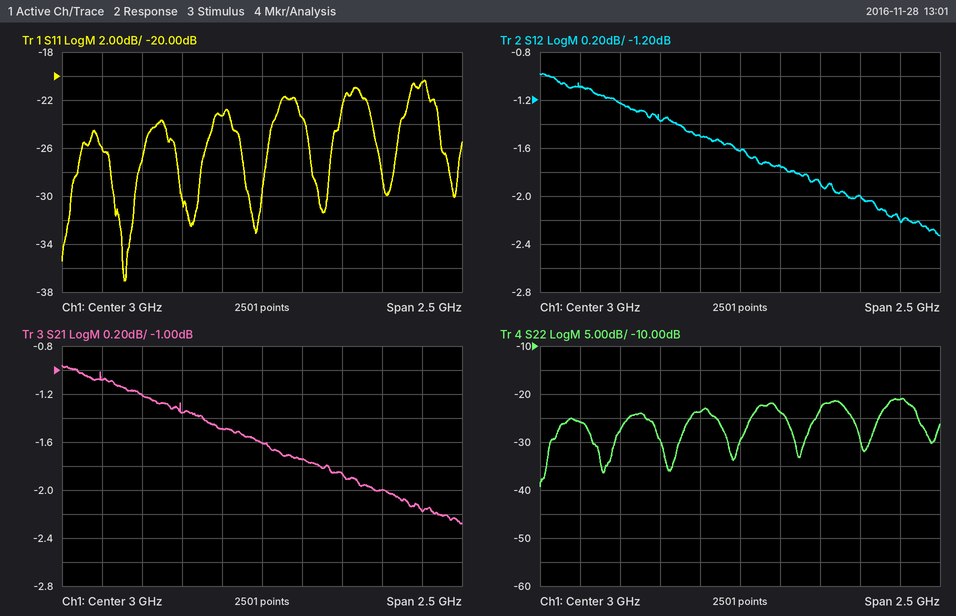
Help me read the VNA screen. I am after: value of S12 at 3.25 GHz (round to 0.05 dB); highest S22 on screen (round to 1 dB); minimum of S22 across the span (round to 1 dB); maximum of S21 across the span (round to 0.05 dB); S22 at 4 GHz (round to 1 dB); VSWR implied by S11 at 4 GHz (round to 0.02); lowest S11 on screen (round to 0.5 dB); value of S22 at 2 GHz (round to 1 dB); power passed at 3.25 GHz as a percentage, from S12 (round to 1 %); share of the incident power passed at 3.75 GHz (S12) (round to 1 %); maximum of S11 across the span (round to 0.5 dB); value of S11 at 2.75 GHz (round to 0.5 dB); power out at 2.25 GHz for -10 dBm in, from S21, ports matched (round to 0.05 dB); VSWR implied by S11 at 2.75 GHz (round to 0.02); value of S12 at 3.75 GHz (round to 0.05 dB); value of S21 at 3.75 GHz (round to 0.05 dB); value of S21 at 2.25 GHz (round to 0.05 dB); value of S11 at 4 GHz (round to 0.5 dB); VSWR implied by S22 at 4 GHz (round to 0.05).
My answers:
-1.75 dB
-21 dB
-39 dB
-0.95 dB
-21 dB
1.20
-37.0 dB
-26 dB
67 %
63 %
-20.5 dB
-23.5 dB
-11.20 dBm
1.14
-2.00 dB
-2.00 dB
-1.20 dB
-20.5 dB
1.20
